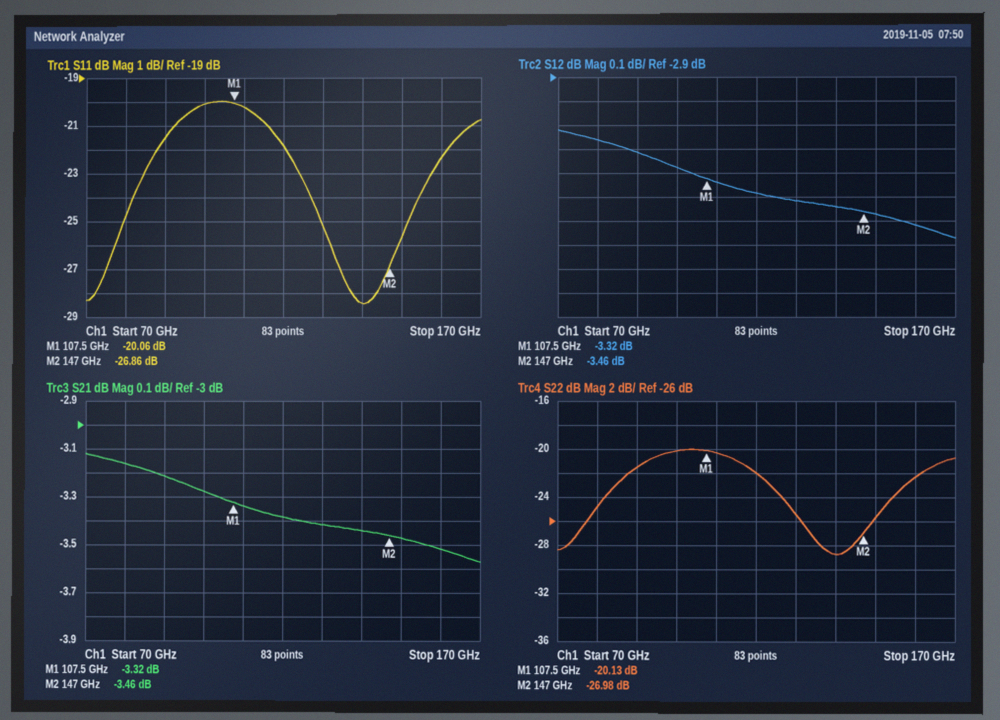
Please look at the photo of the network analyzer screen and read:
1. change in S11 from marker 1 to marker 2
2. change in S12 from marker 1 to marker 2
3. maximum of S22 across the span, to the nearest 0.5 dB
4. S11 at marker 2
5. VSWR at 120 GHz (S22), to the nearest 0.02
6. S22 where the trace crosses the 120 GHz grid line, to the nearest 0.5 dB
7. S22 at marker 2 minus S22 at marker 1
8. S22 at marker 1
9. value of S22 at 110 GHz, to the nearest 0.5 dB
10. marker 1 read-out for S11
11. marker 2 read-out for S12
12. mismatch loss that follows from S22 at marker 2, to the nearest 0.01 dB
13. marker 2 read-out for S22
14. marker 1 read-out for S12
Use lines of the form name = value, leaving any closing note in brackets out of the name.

change in S11 from marker 1 to marker 2 = -6.80 dB
change in S12 from marker 1 to marker 2 = -0.14 dB
maximum of S22 across the span, to the nearest 0.5 dB = -20.0 dB
S11 at marker 2 = -26.86 dB
VSWR at 120 GHz (S22), to the nearest 0.02 = 1.18
S22 where the trace crosses the 120 GHz grid line, to the nearest 0.5 dB = -22.0 dB
S22 at marker 2 minus S22 at marker 1 = -6.85 dB
S22 at marker 1 = -20.13 dB
value of S22 at 110 GHz, to the nearest 0.5 dB = -20.5 dB
marker 1 read-out for S11 = -20.06 dB
marker 2 read-out for S12 = -3.46 dB
mismatch loss that follows from S22 at marker 2, to the nearest 0.01 dB = 0.01 dB
marker 2 read-out for S22 = -26.98 dB
marker 1 read-out for S12 = -3.32 dB
